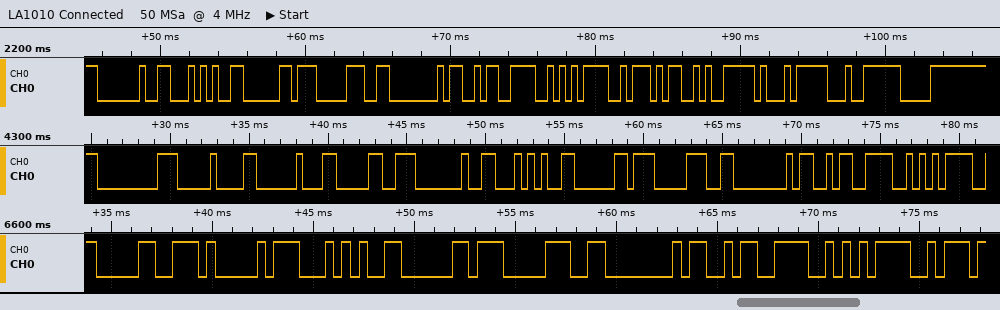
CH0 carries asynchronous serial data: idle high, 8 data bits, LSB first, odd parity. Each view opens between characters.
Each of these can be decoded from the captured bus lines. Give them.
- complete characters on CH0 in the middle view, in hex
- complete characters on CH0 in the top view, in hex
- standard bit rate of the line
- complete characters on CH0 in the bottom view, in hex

00, 10, 20, 30, 40, 54, 60, 70, 80, 9A, AA
40, 54, 60, 70, 80, 9A, AA, BA, CA, D1, E4, F0
2400 baud
30, 41, 54, 60, 70, 80, 9A, AA
